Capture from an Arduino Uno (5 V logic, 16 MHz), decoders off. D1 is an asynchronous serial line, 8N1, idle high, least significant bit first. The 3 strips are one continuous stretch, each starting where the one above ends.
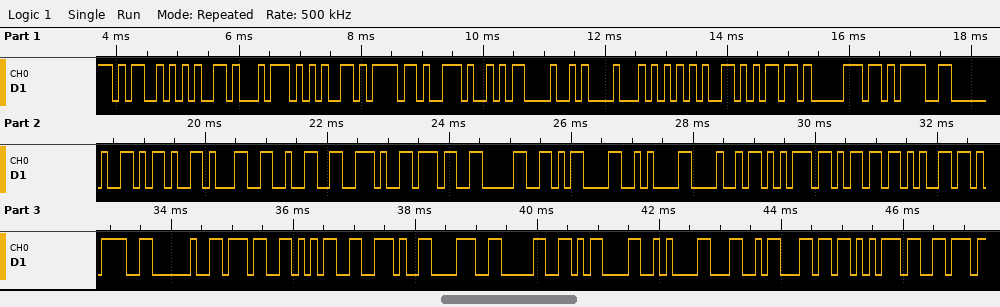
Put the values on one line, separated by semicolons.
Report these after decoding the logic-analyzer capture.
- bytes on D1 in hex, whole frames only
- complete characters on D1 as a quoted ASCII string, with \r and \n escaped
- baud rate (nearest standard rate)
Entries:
4D 65 74 65 6F 2E 0D 0A 54 65 6D 70 3D 20 2D 31 32 2E 37 30 0D 0A 48 75 6D 65 3D 20 37 35 2E 38 30 0D 0A 4C 6C 75 76; "Meteo.\r\nTemp= -12.70\r\nHume= 75.80\r\nLluv"; 9600 baud
